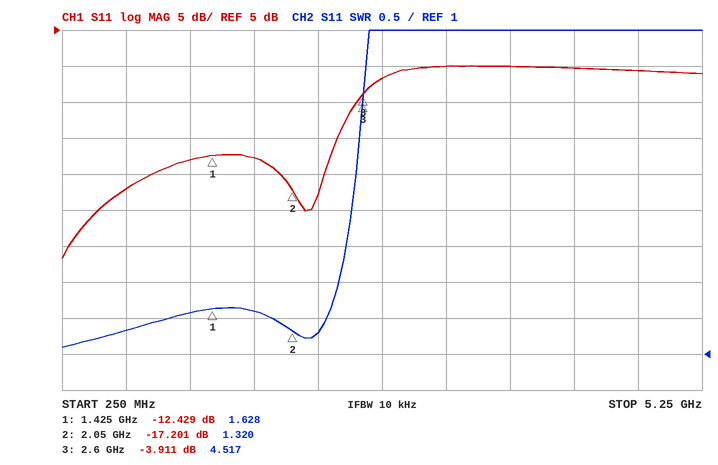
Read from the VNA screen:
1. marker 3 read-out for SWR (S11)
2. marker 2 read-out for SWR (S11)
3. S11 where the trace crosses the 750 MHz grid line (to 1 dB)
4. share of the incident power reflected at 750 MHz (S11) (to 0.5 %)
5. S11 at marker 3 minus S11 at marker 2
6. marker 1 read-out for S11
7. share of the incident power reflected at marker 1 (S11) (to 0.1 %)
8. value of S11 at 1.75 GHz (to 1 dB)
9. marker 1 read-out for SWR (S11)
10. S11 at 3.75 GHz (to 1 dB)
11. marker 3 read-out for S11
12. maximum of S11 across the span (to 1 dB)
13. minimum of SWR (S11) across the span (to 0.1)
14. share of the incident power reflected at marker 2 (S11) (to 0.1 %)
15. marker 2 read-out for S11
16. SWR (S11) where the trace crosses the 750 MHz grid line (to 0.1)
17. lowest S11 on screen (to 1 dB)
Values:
4.517
1.320
-17 dB
2.0 %
13.290 dB
-12.429 dB
5.7 %
-13 dB
1.628
0 dB
-3.911 dB
0 dB
1.1
1.9 %
-17.201 dB
1.3
-27 dB
